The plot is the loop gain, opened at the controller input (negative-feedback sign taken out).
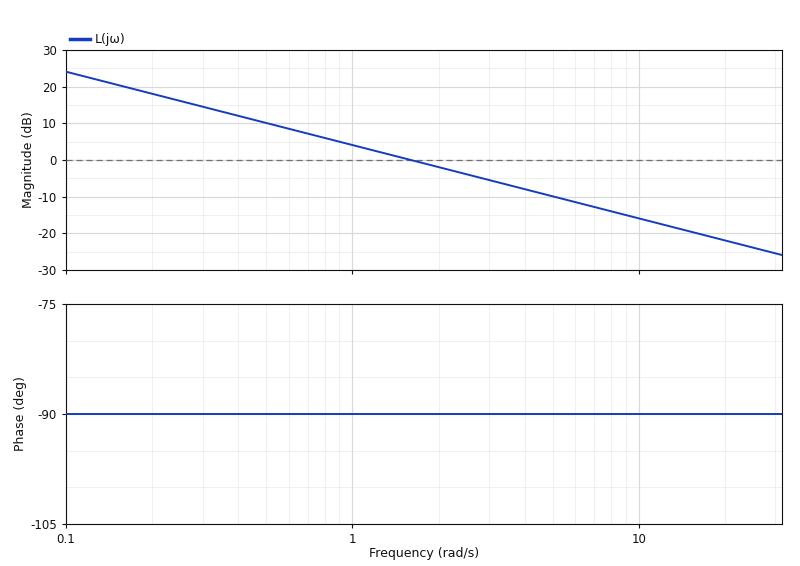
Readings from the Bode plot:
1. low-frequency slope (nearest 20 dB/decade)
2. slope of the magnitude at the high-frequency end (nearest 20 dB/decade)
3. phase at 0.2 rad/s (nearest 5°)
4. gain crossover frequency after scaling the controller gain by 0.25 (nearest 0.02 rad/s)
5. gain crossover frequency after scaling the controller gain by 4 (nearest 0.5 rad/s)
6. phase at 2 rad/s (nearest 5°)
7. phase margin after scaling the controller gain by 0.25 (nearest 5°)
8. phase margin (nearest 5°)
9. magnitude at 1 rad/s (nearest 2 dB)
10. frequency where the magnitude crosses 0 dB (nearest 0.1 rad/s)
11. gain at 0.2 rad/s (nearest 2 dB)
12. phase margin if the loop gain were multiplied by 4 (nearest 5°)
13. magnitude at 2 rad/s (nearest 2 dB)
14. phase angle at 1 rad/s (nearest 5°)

-20 dB/decade
-20 dB/decade
-90°
0.40 rad/s
6.5 rad/s
-90°
90°
90°
4 dB
1.6 rad/s
18 dB
90°
-2 dB
-90°
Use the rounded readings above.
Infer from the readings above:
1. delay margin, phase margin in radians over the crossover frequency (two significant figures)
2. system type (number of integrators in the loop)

0.98 s
1
